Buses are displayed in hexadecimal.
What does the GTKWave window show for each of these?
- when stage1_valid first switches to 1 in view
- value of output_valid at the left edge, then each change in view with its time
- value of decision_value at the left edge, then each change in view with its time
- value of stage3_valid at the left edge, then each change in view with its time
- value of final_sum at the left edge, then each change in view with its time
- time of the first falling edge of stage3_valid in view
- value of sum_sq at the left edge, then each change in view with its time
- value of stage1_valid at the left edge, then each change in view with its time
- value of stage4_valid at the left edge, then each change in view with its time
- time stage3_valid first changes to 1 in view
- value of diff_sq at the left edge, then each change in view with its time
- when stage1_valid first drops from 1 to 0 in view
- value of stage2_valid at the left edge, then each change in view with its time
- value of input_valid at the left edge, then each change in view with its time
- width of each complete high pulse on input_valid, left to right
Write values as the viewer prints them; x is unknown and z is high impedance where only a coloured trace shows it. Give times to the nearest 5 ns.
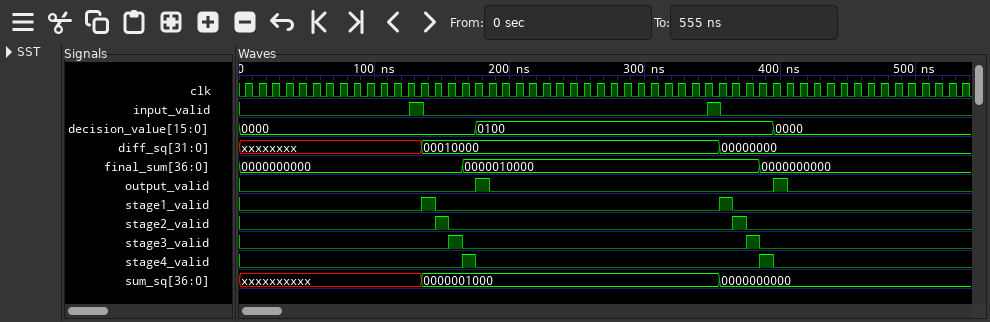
135 ns
0, 1 at 175 ns, 0 at 185 ns, 1 at 395 ns, 0 at 405 ns
0000, 0100 at 175 ns, 0000 at 395 ns
0, 1 at 155 ns, 0 at 165 ns, 1 at 375 ns, 0 at 385 ns
0000000000, 0000010000 at 165 ns, 0000000000 at 385 ns
165 ns
xxxxxxxxxx, 0000001000 at 135 ns, 0000000000 at 355 ns
0, 1 at 135 ns, 0 at 145 ns, 1 at 355 ns, 0 at 365 ns
0, 1 at 165 ns, 0 at 175 ns, 1 at 385 ns, 0 at 395 ns
155 ns
xxxxxxxx, 00010000 at 135 ns, 00000000 at 355 ns
145 ns
0, 1 at 145 ns, 0 at 155 ns, 1 at 365 ns, 0 at 375 ns
0, 1 at 125 ns, 0 at 135 ns, 1 at 345 ns, 0 at 355 ns
10 ns, 10 ns
